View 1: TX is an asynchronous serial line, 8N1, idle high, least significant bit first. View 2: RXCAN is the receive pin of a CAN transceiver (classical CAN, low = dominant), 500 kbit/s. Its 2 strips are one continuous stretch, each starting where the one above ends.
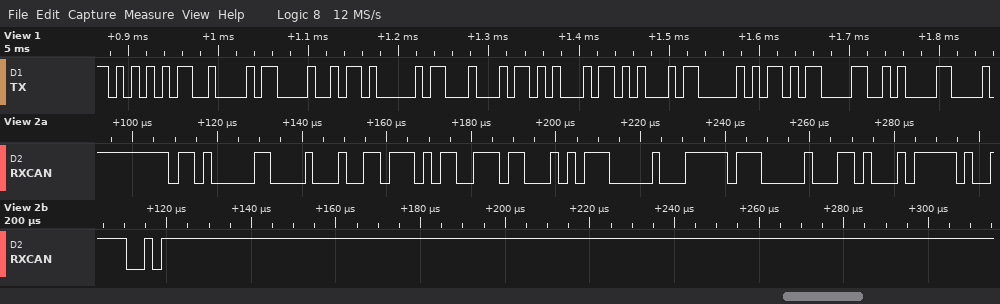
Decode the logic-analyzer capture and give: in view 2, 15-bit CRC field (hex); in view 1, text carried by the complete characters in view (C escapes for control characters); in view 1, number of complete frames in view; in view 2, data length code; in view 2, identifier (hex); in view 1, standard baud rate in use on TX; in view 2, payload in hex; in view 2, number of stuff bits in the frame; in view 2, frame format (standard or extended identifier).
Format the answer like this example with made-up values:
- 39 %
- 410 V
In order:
- 0x3F3C
- "UBHADEEP\r\n"
- 10
- 8
- 0x682
- 115200 baud
- 9B AC EC 57 00 FF 00 D1
- 5
- standard
